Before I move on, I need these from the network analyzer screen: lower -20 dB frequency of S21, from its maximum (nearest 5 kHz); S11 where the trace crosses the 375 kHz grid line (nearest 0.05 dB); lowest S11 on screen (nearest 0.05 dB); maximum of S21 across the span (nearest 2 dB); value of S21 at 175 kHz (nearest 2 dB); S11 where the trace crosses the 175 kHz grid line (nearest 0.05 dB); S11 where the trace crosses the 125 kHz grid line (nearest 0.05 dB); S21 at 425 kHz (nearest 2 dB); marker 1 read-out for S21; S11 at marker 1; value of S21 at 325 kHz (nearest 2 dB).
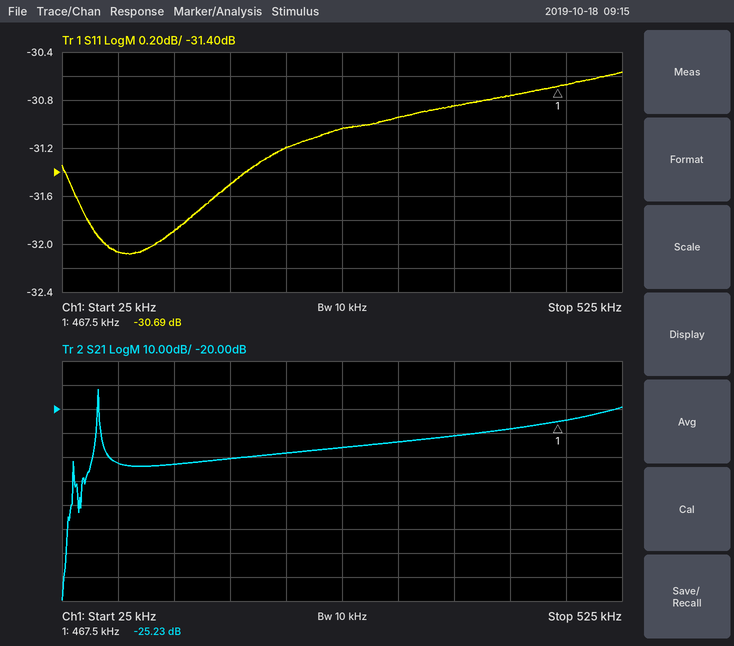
55 kHz
-30.85 dB
-32.10 dB
-12 dB
-40 dB
-31.50 dB
-31.90 dB
-28 dB
-25.23 dB
-30.69 dB
-34 dB
